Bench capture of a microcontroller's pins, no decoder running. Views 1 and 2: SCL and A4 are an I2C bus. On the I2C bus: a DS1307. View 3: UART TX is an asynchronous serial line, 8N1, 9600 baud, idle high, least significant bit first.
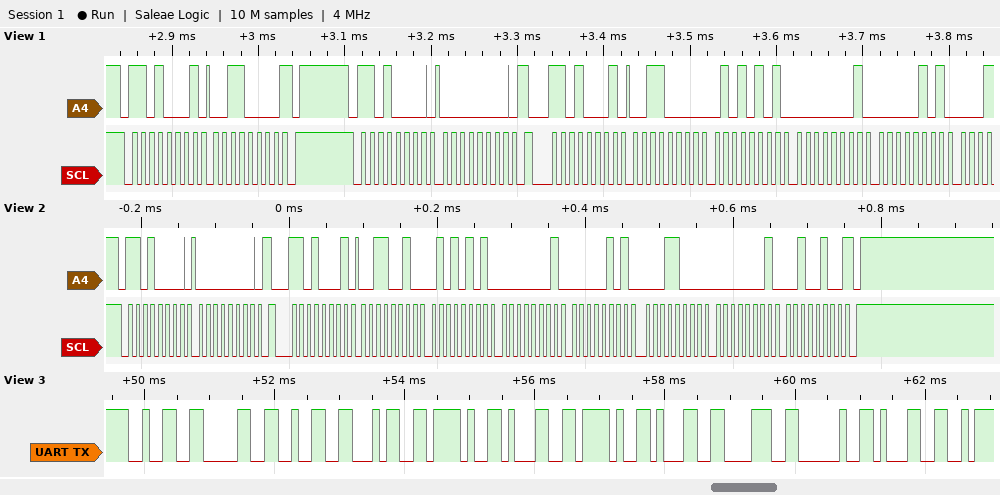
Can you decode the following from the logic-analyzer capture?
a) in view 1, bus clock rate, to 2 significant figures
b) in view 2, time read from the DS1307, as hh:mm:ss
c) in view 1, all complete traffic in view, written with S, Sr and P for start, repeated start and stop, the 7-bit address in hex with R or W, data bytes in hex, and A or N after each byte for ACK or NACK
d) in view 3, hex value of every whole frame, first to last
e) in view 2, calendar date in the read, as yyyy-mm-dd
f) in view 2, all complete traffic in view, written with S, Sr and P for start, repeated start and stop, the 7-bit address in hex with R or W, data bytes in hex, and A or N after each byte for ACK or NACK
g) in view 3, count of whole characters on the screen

100 kHz
01:55:32
S 68R A 30 N P S 68W A 00 A Sr 68R A 30 A 55 A 01 A 05 A
32 30 32 34 2F 31 2F 31 38 20 31
2024-01-18
S 68W A 00 A Sr 68R A 32 A 55 A 01 A 05 A 18 A 01 A 24 N P
11
